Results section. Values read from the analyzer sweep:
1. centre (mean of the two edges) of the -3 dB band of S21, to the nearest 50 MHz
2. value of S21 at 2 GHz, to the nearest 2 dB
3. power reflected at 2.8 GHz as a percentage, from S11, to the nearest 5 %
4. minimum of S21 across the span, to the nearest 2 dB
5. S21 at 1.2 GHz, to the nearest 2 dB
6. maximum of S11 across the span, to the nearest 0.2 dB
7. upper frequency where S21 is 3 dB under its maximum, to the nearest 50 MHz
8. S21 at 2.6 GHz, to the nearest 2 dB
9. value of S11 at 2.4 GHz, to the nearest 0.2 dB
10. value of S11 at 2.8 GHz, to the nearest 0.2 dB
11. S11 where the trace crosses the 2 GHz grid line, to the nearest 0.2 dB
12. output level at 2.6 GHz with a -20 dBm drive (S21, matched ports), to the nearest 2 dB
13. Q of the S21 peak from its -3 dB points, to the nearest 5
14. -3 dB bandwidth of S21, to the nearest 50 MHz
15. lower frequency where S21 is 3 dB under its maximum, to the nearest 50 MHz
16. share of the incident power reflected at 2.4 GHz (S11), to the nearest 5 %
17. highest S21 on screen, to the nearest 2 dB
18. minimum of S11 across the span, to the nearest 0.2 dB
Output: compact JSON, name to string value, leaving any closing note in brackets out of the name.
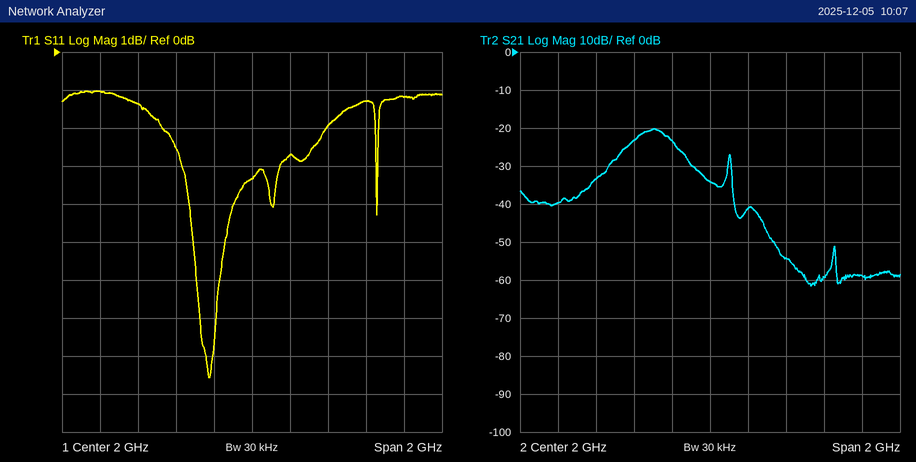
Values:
{"centre (mean of the two edges) of the -3 dB band of S21, to the nearest 50 MHz": "1.70 GHz", "value of S21 at 2 GHz, to the nearest 2 dB": "-34 dB", "power reflected at 2.8 GHz as a percentage, from S11, to the nearest 5 %": "75 %", "minimum of S21 across the span, to the nearest 2 dB": "-62 dB", "S21 at 1.2 GHz, to the nearest 2 dB": "-40 dB", "maximum of S11 across the span, to the nearest 0.2 dB": "-1.0 dB", "upper frequency where S21 is 3 dB under its maximum, to the nearest 50 MHz": "1.80 GHz", "S21 at 2.6 GHz, to the nearest 2 dB": "-60 dB", "value of S11 at 2.4 GHz, to the nearest 0.2 dB": "-2.0 dB", "value of S11 at 2.8 GHz, to the nearest 0.2 dB": "-1.2 dB", "S11 where the trace crosses the 2 GHz grid line, to the nearest 0.2 dB": "-3.4 dB", "output level at 2.6 GHz with a -20 dBm drive (S21, matched ports), to the nearest 2 dB": "-80 dBm", "Q of the S21 peak from its -3 dB points, to the nearest 5": "10", "-3 dB bandwidth of S21, to the nearest 50 MHz": "200 MHz", "lower frequency where S21 is 3 dB under its maximum, to the nearest 50 MHz": "1.60 GHz", "share of the incident power reflected at 2.4 GHz (S11), to the nearest 5 %": "65 %", "highest S21 on screen, to the nearest 2 dB": "-20 dB", "minimum of S11 across the span, to the nearest 0.2 dB": "-8.6 dB"}
